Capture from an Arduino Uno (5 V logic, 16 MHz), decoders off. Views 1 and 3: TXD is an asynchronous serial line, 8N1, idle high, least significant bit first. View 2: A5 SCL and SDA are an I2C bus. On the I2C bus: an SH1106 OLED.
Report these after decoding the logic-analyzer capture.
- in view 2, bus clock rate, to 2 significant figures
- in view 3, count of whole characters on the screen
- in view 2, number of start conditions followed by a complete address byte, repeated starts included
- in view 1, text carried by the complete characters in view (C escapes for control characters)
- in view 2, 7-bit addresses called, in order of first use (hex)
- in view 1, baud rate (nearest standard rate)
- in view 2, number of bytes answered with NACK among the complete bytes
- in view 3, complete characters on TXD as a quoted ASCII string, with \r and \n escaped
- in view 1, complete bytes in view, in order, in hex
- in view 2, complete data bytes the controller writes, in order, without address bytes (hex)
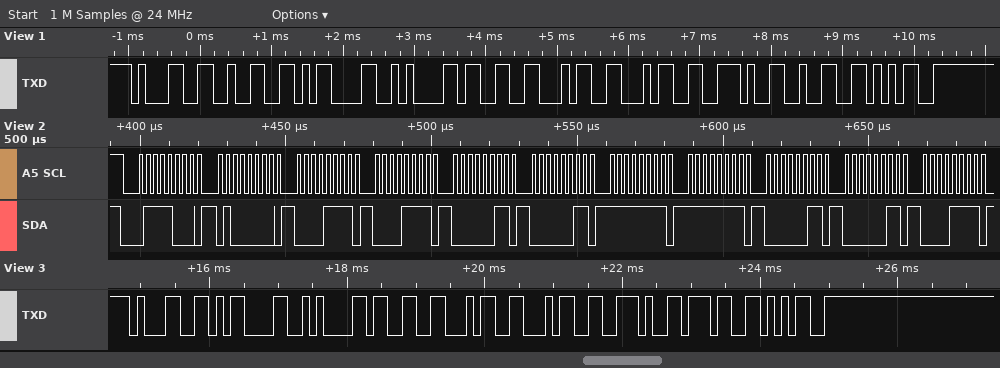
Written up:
400 kHz
9
1
"12\r\n344.25"
0x3C
9600 baud
0
"1\r\n344.75"
31 32 0D 0A 33 34 34 2E 32 35
40 0F 0F 03 03 FF FF 03 03 0F
